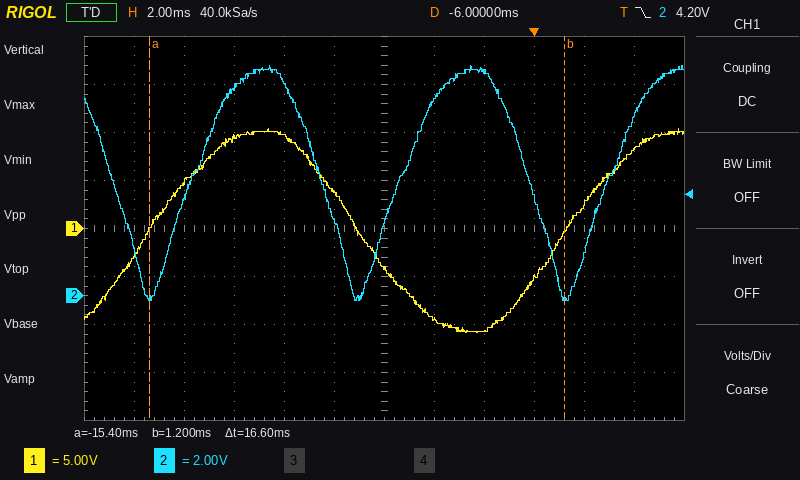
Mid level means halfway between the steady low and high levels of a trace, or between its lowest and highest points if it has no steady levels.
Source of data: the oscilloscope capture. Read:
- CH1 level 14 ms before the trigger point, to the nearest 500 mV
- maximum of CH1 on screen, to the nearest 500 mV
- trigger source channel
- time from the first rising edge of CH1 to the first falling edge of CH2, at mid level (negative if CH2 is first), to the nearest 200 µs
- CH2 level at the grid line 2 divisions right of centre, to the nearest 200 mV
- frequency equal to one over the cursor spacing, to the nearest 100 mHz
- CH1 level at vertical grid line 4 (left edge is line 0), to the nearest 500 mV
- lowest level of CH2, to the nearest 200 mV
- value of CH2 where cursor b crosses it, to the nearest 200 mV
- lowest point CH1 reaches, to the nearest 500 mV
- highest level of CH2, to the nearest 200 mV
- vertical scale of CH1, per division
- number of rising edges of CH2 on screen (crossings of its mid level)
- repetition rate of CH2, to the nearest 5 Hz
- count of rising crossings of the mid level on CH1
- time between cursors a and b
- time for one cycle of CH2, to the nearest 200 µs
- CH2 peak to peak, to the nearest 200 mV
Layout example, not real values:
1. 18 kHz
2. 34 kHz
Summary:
1. 5.0 V
2. 10.5 V
3. CH2
4. -1.4 ms
5. 9.4 V
6. 60.2 Hz
7. 9.5 V
8. -200 mV
9. 0.0 V
10. -11.0 V
11. 9.6 V
12. 5 V
13. 3
14. 120 Hz
15. 2
16. 16.6 ms
17. 8.4 ms
18. 9.8 V
